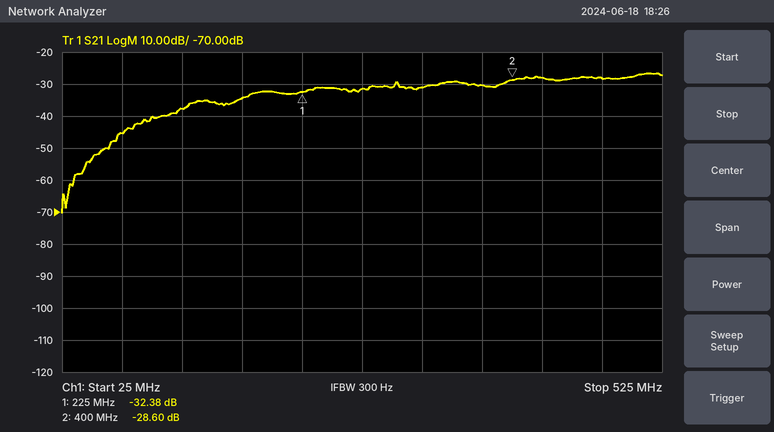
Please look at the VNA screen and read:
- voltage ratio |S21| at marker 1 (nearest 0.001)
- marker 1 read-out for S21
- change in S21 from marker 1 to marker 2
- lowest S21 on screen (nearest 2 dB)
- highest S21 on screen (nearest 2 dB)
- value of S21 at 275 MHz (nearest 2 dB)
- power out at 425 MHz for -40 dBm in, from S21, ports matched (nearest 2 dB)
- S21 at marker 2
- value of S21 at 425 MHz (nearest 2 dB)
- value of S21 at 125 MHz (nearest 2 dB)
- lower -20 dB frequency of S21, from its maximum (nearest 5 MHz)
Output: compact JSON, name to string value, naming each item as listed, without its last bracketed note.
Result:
{"voltage ratio |S21| at marker 1": "0.024", "marker 1 read-out for S21": "-32.38 dB", "change in S21 from marker 1 to marker 2": "3.78 dB", "lowest S21 on screen": "-70 dB", "highest S21 on screen": "-26 dB", "value of S21 at 275 MHz": "-32 dB", "power out at 425 MHz for -40 dBm in, from S21, ports matched": "-68 dBm", "S21 at marker 2": "-28.60 dB", "value of S21 at 425 MHz": "-28 dB", "value of S21 at 125 MHz": "-38 dB", "lower -20 dB frequency of S21, from its maximum": "70 MHz"}
